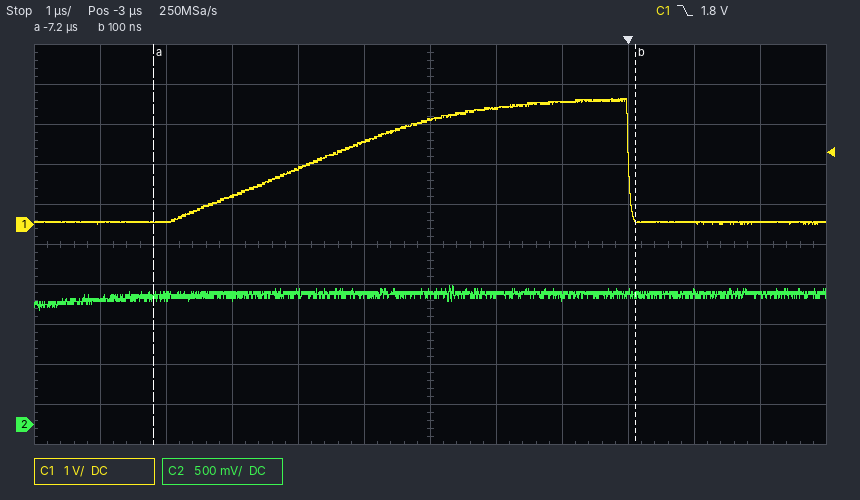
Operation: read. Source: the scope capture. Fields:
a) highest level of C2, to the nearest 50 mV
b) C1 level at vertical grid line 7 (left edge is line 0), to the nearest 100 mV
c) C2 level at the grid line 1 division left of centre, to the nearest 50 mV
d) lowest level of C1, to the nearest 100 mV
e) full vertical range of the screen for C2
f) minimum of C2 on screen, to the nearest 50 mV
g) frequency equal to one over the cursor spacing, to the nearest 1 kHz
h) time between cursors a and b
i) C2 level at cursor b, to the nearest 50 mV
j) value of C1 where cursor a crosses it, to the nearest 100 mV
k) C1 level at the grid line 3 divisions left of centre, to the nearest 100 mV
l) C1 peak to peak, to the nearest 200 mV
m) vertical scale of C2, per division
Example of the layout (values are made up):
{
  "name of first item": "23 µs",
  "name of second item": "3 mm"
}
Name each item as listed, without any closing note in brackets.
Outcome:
{
  "highest level of C2, to the nearest 50 mV": "1.75 V",
  "C1 level at vertical grid line 7 (left edge is line 0), to the nearest 100 mV": "2.9 V",
  "C2 level at the grid line 1 division left of centre, to the nearest 50 mV": "1.60 V",
  "lowest level of C1, to the nearest 100 mV": "0.0 V",
  "full vertical range of the screen for C2": "5 V",
  "minimum of C2 on screen, to the nearest 50 mV": "1.40 V",
  "frequency equal to one over the cursor spacing, to the nearest 1 kHz": "137 kHz",
  "time between cursors a and b": "7.3 µs",
  "C2 level at cursor b, to the nearest 50 mV": "1.60 V",
  "value of C1 where cursor a crosses it, to the nearest 100 mV": "100 mV",
  "C1 level at the grid line 3 divisions left of centre, to the nearest 100 mV": "700 mV",
  "C1 peak to peak, to the nearest 200 mV": "3.2 V",
  "vertical scale of C2, per division": "500 mV"
}
